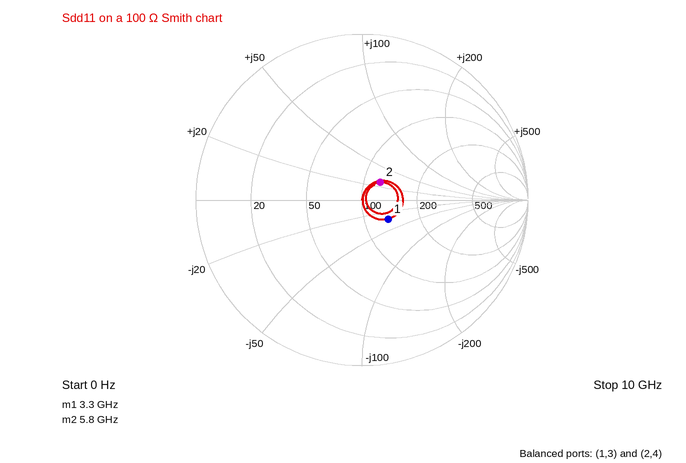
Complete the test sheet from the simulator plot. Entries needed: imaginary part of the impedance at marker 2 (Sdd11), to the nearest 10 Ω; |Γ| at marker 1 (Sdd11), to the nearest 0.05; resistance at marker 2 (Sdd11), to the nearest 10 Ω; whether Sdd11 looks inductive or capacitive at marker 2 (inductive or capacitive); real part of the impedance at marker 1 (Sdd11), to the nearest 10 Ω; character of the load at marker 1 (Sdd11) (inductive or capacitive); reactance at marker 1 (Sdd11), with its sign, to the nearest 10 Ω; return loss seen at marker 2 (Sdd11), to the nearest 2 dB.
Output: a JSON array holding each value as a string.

["+30 Ω", "0.20", "120 Ω", "inductive", "130 Ω", "capacitive", "-30 Ω", "16 dB"]
